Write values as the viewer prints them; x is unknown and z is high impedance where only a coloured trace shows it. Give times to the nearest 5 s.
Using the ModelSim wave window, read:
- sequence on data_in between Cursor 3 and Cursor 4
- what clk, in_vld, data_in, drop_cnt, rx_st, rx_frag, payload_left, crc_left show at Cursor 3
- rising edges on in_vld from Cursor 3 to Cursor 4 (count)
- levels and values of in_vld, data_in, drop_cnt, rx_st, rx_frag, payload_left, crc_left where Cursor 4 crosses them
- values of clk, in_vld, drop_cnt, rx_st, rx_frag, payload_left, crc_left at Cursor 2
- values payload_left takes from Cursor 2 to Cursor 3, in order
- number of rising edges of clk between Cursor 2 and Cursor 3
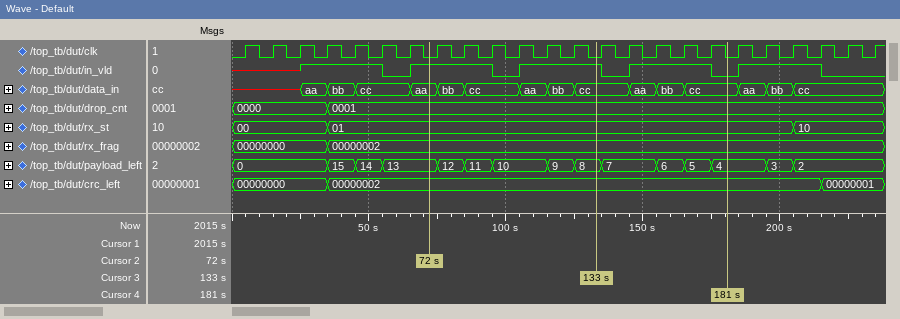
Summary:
cc, aa, bb, cc
clk=0, in_vld=1, data_in=cc, drop_cnt=0001, rx_st=01, rx_frag=00000002, payload_left=8, crc_left=00000002
1
in_vld=0, data_in=cc, drop_cnt=0001, rx_st=01, rx_frag=00000002, payload_left=4, crc_left=00000002
clk=0, in_vld=1, drop_cnt=0001, rx_st=01, rx_frag=00000002, payload_left=13, crc_left=00000002
13, 12, 11, 10, 9, 8
6
